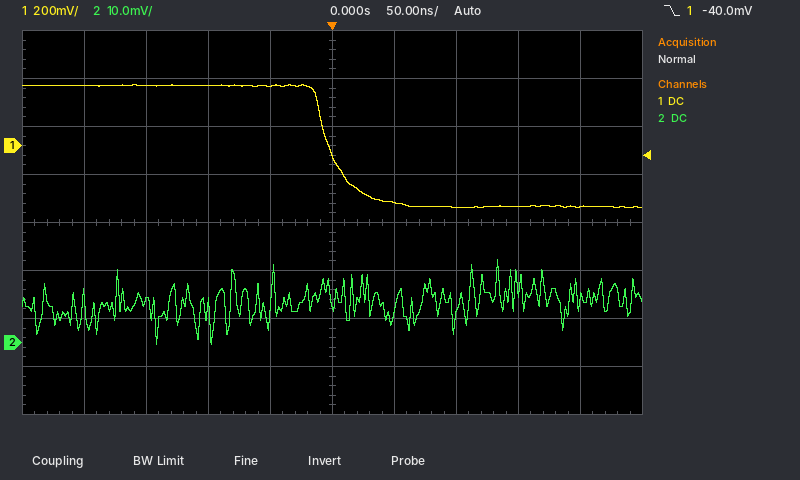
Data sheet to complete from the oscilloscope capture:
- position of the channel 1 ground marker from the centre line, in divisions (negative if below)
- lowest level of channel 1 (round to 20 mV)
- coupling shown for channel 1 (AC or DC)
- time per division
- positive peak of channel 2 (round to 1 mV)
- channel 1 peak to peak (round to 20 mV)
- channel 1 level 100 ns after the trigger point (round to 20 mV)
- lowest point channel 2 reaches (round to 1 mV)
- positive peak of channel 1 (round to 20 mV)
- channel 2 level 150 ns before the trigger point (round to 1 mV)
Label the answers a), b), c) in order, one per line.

a) +1.6 div
b) -260 mV
c) DC
d) 50 ns
e) 17 mV
f) 520 mV
g) -260 mV
h) 0 mV
i) 260 mV
j) 8 mV
